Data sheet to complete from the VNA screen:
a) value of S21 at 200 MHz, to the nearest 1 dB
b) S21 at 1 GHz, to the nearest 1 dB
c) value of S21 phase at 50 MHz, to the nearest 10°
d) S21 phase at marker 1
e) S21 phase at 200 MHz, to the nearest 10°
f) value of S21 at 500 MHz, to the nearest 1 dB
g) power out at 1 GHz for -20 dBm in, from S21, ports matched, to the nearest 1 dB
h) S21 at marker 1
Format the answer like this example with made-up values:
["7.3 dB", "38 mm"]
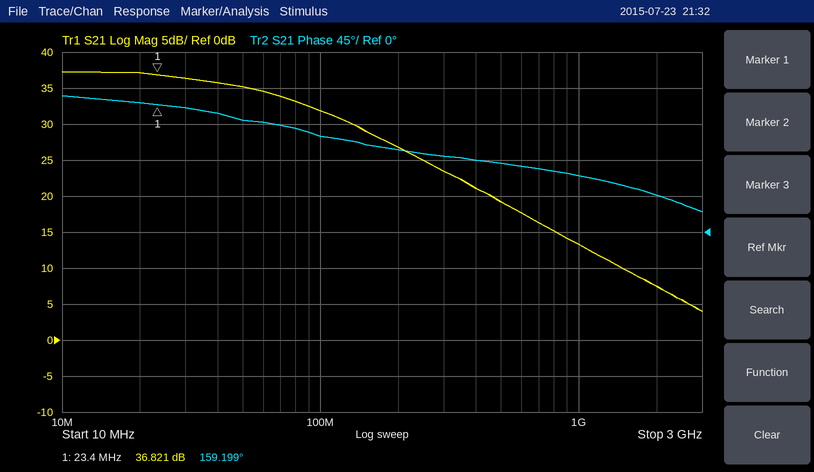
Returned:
["27 dB", "13 dB", "140°", "159.199°", "100°", "19 dB", "-7 dBm", "36.821 dB"]
